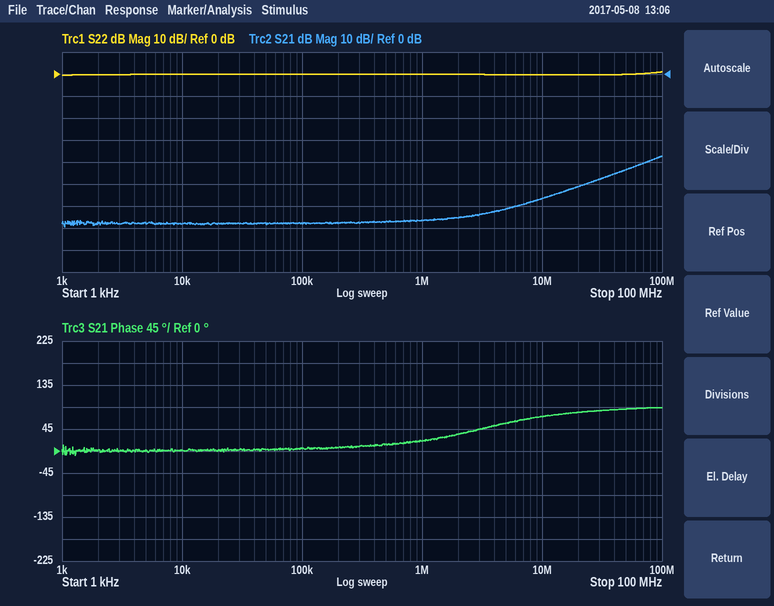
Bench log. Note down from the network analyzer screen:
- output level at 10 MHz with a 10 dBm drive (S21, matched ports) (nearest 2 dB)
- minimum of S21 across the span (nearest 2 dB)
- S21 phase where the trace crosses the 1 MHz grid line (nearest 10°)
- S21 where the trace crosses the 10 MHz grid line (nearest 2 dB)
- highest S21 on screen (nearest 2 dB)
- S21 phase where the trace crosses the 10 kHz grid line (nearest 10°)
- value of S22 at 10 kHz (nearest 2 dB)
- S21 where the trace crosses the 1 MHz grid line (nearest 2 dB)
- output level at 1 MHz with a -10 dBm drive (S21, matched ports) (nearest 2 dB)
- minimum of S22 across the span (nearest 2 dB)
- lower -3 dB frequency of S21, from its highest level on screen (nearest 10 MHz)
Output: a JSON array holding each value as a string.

["-46 dBm", "-70 dB", "20°", "-56 dB", "-38 dB", "0°", "0 dB", "-66 dB", "-76 dBm", "0 dB", "70 MHz"]
